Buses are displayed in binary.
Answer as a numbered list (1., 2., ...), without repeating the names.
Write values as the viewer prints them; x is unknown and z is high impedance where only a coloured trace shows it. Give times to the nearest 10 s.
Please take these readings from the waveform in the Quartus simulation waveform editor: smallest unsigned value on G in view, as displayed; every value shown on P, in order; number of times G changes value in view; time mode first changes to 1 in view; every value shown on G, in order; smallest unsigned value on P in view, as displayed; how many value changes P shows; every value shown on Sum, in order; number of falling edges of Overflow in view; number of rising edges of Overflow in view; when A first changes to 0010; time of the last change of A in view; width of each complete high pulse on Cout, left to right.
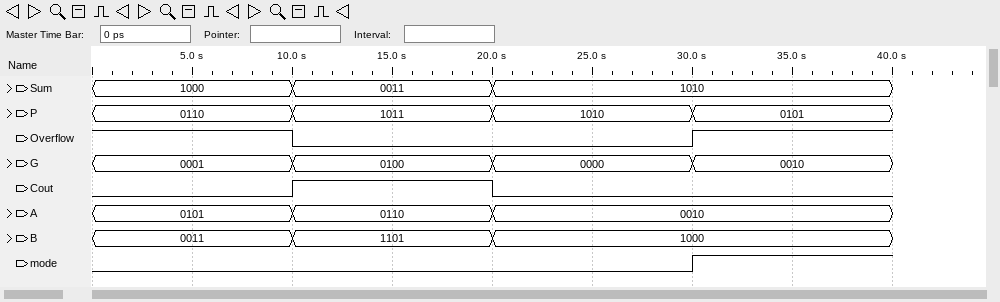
1. 0000
2. 0110, 1011, 1010, 0101
3. 3
4. 30 s
5. 0001, 0100, 0000, 0010
6. 0101
7. 3
8. 1000, 0011, 1010
9. 1
10. 1
11. 20 s
12. 20 s
13. 10 s
